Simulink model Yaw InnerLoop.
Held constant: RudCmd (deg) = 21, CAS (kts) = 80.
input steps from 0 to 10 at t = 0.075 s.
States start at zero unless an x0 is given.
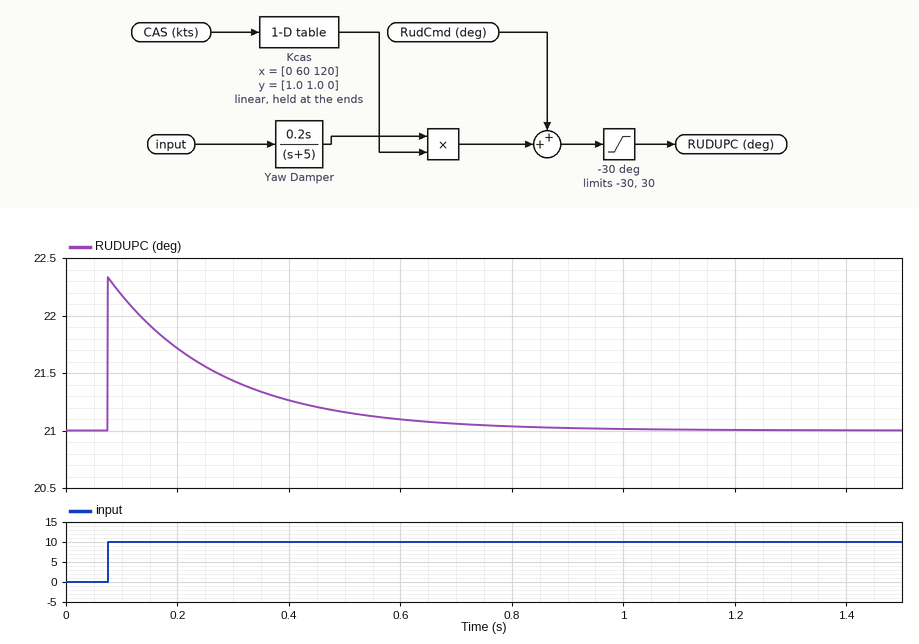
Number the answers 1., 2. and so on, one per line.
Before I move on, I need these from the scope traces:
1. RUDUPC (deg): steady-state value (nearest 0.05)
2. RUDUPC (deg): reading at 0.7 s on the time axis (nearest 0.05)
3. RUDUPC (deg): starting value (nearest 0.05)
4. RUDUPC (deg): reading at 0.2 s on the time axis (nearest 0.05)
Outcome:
1. 21.00
2. 21.05
3. 21.00
4. 21.70
